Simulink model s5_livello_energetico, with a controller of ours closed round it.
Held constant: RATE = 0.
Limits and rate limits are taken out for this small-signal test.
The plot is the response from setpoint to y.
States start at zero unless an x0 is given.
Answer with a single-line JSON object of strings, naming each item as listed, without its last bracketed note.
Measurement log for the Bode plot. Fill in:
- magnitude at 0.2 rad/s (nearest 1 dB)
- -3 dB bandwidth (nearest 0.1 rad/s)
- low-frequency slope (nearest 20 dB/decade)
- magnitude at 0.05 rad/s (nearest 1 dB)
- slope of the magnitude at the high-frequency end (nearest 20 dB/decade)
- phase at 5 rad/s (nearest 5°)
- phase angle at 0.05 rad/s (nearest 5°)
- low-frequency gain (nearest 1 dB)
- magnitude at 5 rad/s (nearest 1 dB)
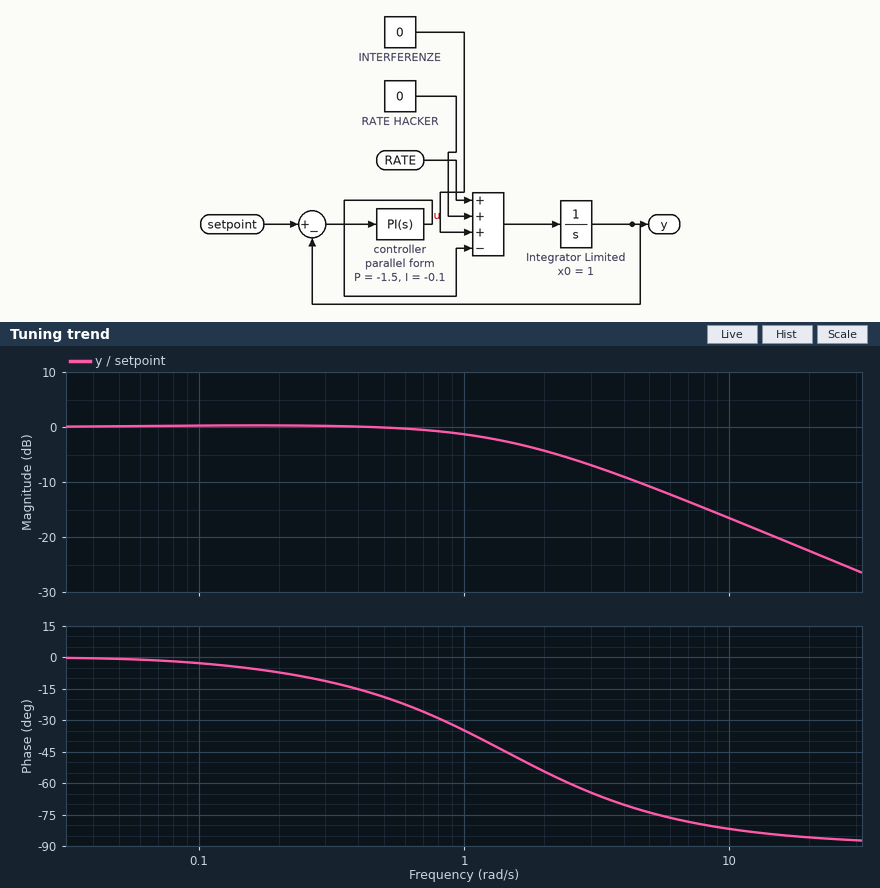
{"magnitude at 0.2 rad/s": "0 dB", "-3 dB bandwidth": "1.5 rad/s", "low-frequency slope": "0 dB/decade", "magnitude at 0.05 rad/s": "0 dB", "slope of the magnitude at the high-frequency end": "-20 dB/decade", "phase at 5 rad/s": "-75°", "phase angle at 0.05 rad/s": "0°", "low-frequency gain": "0 dB", "magnitude at 5 rad/s": "-11 dB"}
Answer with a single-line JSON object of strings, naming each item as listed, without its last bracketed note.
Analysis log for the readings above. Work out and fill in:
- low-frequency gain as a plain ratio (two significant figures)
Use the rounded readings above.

{"low-frequency gain as a plain ratio": "1.0"}
